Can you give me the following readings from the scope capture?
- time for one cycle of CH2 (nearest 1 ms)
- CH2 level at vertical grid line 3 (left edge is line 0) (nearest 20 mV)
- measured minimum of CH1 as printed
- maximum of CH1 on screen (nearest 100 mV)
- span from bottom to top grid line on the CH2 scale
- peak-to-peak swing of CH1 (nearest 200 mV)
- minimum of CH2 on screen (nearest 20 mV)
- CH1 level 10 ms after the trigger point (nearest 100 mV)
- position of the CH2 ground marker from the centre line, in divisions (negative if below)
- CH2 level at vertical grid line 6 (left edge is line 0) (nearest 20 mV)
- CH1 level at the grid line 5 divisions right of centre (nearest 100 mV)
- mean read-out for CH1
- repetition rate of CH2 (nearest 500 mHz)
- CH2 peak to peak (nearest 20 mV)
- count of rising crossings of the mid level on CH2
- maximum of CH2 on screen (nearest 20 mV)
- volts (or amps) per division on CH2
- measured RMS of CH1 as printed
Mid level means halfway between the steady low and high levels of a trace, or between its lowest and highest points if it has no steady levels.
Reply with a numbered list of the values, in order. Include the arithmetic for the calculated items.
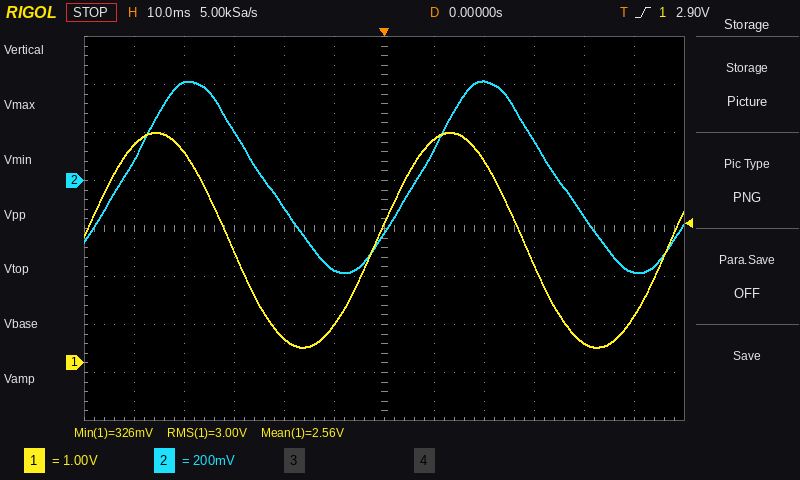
1. 59 ms
2. 200 mV
3. 326 mV
4. 4.8 V
5. 1.6 V
6. 4.4 V
7. -380 mV
8. 4.7 V
9. +1.0 div
10. -220 mV
11. 1.0 V
12. 2.56 V
13. 1 / 59 ms ≈ 16.9 Hz, so 17.0 Hz to the nearest 500 mHz
14. 420 mV − (-380 mV) = 800 mV
15. 2
16. 420 mV
17. 200 mV
18. 3.00 V
